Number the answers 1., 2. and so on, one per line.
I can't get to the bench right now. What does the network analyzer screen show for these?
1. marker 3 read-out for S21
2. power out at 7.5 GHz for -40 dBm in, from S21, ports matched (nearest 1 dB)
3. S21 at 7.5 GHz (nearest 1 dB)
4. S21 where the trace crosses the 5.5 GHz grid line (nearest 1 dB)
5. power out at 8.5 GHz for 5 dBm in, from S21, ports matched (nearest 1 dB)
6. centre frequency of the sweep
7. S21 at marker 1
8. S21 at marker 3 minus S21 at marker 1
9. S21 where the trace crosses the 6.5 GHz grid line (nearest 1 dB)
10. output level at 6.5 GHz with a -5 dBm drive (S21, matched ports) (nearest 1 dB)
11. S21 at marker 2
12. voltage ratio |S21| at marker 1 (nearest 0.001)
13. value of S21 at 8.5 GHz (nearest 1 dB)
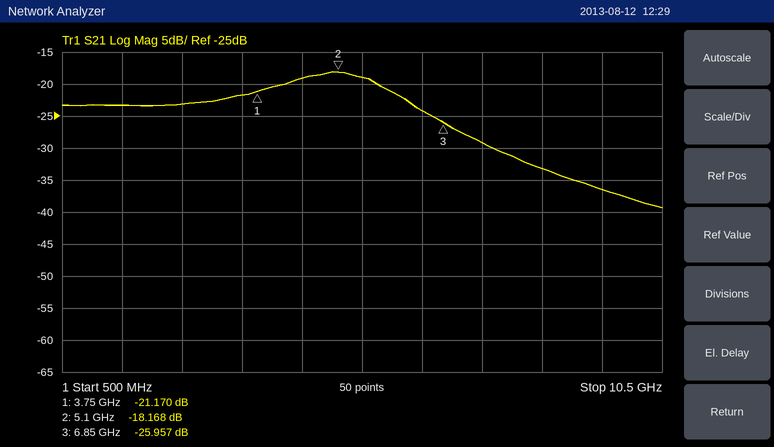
1. -25.957 dB
2. -69 dBm
3. -29 dB
4. -19 dB
5. -28 dBm
6. 5.5 GHz
7. -21.170 dB
8. -4.787 dB
9. -24 dB
10. -29 dBm
11. -18.168 dB
12. 0.087
13. -33 dB
